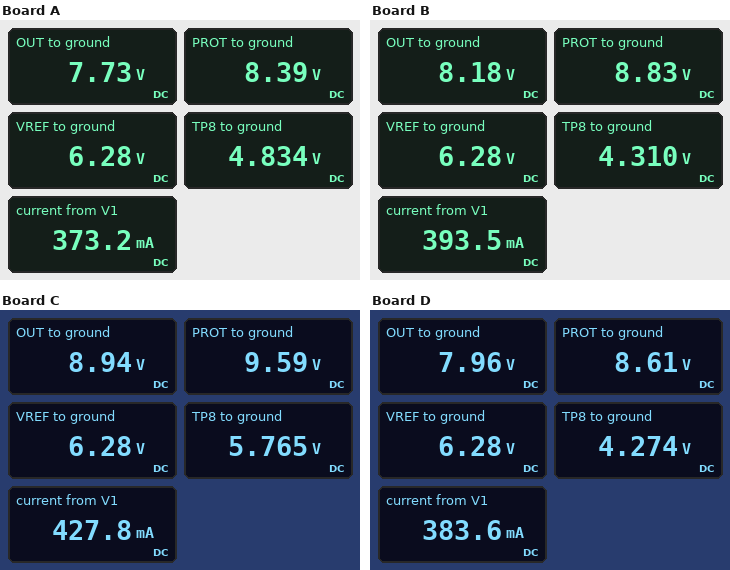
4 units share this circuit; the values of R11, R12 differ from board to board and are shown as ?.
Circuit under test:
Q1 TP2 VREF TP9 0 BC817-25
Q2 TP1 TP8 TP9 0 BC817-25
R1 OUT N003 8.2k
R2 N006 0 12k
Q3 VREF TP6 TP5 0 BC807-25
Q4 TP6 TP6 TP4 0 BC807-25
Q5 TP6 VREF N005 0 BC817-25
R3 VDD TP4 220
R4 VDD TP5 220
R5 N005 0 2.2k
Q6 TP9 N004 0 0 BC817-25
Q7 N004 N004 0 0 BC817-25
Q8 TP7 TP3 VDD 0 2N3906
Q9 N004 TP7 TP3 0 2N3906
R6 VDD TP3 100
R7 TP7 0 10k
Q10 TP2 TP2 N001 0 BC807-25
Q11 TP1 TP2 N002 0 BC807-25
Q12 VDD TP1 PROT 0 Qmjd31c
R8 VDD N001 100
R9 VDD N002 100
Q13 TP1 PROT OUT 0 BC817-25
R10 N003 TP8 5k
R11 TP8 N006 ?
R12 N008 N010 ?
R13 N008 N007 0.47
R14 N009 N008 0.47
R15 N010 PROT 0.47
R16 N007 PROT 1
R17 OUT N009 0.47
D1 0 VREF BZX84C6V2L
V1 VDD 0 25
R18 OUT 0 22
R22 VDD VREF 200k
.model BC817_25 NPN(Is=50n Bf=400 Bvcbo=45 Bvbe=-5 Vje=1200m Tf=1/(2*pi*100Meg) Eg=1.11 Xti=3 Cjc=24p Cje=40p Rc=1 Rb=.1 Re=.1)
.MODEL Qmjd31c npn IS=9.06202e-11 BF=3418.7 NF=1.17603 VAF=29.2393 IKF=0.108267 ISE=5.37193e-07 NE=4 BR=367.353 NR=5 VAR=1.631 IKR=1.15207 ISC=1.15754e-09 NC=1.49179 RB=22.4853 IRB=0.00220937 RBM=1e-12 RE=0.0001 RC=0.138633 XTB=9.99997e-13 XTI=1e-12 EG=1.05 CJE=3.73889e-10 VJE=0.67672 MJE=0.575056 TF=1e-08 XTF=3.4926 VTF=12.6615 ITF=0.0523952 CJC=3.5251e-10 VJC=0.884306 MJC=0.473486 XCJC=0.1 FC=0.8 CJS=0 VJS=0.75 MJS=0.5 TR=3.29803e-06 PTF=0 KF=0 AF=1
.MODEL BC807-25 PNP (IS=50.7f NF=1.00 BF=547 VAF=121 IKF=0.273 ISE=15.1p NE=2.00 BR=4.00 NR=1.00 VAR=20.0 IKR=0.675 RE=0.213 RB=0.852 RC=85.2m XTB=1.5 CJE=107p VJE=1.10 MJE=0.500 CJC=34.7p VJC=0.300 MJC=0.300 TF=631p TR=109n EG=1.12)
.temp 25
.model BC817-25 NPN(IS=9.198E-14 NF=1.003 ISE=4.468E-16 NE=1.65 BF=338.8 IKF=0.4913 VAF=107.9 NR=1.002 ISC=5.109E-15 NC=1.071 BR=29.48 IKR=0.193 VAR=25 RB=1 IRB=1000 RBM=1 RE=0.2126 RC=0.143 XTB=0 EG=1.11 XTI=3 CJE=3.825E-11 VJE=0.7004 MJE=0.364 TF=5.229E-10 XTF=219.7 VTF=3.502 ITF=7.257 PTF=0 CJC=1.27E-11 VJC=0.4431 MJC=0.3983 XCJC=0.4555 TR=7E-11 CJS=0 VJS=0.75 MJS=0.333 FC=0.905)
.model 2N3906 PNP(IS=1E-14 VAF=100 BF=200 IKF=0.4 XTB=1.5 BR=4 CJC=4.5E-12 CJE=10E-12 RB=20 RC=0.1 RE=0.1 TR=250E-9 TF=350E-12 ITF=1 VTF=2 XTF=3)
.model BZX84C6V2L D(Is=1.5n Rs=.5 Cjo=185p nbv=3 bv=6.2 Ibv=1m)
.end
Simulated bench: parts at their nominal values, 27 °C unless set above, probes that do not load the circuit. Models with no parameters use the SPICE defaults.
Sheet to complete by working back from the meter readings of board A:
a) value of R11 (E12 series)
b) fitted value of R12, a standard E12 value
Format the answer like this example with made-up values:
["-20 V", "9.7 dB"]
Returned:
["10 kΩ", "2.2 Ω"]
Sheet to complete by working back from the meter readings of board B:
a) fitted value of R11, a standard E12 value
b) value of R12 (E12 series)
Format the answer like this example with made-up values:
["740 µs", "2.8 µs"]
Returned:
["2.7 kΩ", "1.5 Ω"]
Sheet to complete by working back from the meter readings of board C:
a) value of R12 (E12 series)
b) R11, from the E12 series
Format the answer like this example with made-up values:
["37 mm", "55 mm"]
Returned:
["0.82 Ω", "12 kΩ"]
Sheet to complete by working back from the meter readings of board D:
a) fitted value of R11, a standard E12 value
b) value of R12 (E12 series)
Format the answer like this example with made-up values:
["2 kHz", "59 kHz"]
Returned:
["3.3 kΩ", "1.8 Ω"]
